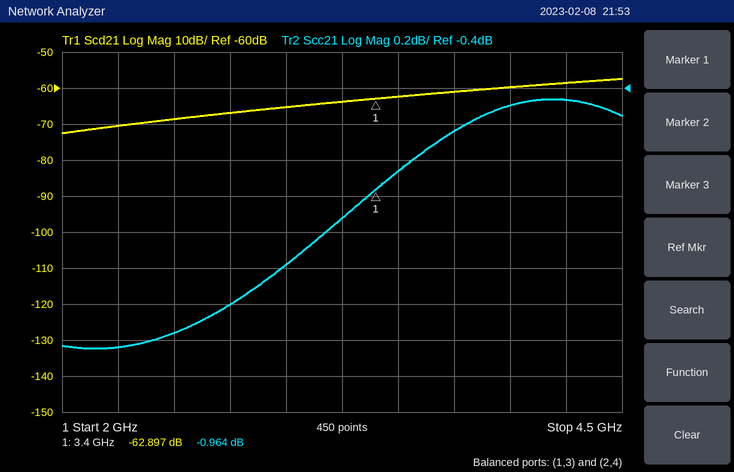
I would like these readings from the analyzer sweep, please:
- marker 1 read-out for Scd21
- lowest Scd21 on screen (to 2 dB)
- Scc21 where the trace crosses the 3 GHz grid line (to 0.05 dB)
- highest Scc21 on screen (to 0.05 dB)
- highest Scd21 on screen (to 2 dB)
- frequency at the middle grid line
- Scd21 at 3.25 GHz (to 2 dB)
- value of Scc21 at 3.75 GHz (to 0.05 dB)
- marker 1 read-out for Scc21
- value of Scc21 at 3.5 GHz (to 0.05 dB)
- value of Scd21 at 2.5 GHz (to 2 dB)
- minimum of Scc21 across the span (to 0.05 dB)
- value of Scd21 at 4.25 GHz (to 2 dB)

-62.897 dB
-72 dB
-1.40 dB
-0.45 dB
-58 dB
3.25 GHz
-64 dB
-0.65 dB
-0.964 dB
-0.85 dB
-68 dB
-1.85 dB
-58 dB
